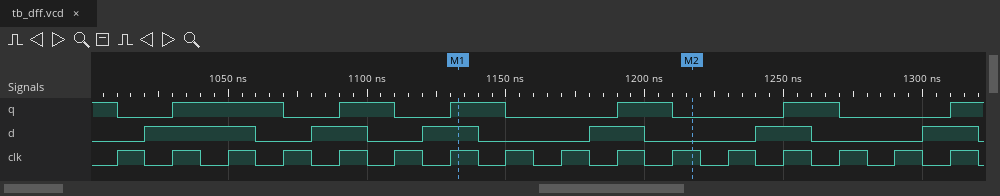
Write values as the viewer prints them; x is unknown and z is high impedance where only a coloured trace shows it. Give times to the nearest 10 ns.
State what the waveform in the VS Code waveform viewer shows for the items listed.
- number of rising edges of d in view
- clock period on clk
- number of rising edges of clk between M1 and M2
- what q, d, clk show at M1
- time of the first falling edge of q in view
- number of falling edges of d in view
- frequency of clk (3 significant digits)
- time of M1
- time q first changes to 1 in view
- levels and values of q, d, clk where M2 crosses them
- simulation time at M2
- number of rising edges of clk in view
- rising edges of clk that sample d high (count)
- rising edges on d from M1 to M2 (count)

6
20 ns
4
q=1, d=1, clk=1
1010 ns
6
50.0 MHz
1130 ns
1030 ns
q=0, d=0, clk=1
1220 ns
16
7
1
